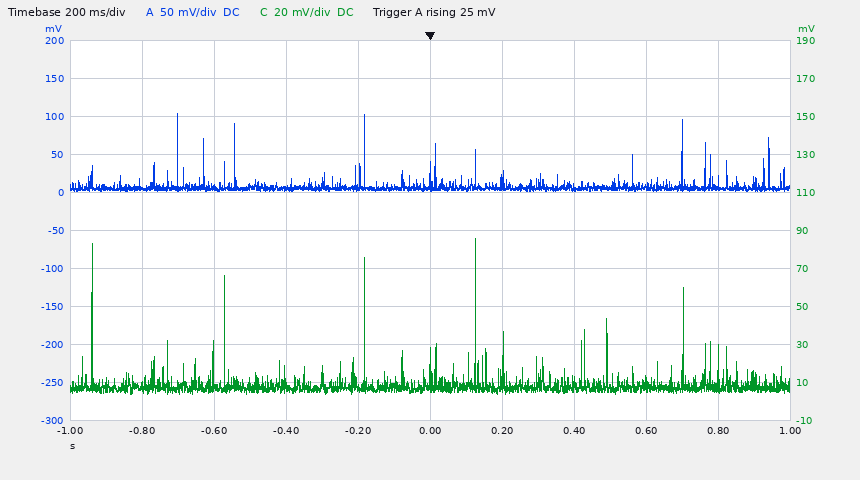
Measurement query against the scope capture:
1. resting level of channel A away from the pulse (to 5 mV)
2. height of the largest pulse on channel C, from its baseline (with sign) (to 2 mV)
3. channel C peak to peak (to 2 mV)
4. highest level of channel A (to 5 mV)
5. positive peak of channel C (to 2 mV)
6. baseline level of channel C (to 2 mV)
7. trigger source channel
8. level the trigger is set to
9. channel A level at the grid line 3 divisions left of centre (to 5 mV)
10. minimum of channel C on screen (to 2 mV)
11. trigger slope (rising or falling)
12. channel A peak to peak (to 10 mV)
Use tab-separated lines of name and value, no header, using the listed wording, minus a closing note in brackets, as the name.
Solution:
resting level of channel A away from the pulse	5 mV
height of the largest pulse on channel C, from its baseline (with sign)	+78 mV
channel C peak to peak	82 mV
highest level of channel A	105 mV
positive peak of channel C	86 mV
baseline level of channel C	8 mV
trigger source channel	channel A
level the trigger is set to	25 mV
channel A level at the grid line 3 divisions left of centre	10 mV
minimum of channel C on screen	4 mV
trigger slope	rising
channel A peak to peak	100 mV
